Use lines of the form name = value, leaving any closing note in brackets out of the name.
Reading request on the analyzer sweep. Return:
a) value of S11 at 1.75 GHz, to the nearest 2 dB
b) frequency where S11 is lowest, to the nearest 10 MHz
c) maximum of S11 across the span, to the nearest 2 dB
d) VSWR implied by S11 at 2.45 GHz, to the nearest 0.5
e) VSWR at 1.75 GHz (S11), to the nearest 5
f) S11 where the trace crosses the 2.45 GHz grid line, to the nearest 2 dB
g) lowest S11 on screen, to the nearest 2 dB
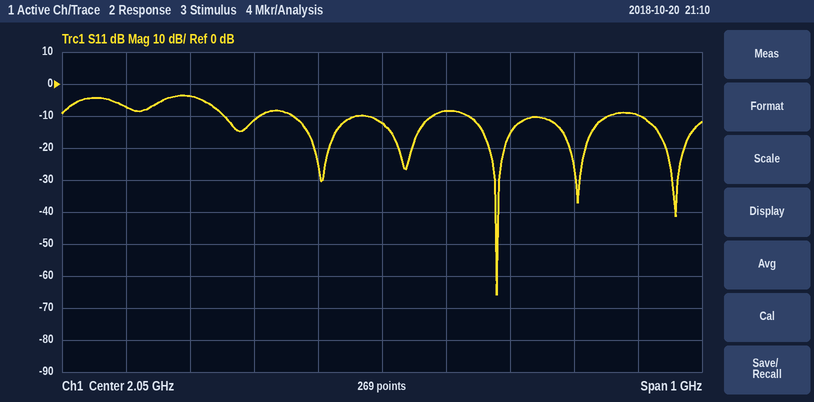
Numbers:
value of S11 at 1.75 GHz, to the nearest 2 dB = -4 dB
frequency where S11 is lowest, to the nearest 10 MHz = 2.23 GHz
maximum of S11 across the span, to the nearest 2 dB = -4 dB
VSWR implied by S11 at 2.45 GHz, to the nearest 0.5 = 2.0
VSWR at 1.75 GHz (S11), to the nearest 5 = 5
S11 where the trace crosses the 2.45 GHz grid line, to the nearest 2 dB = -10 dB
lowest S11 on screen, to the nearest 2 dB = -66 dB
